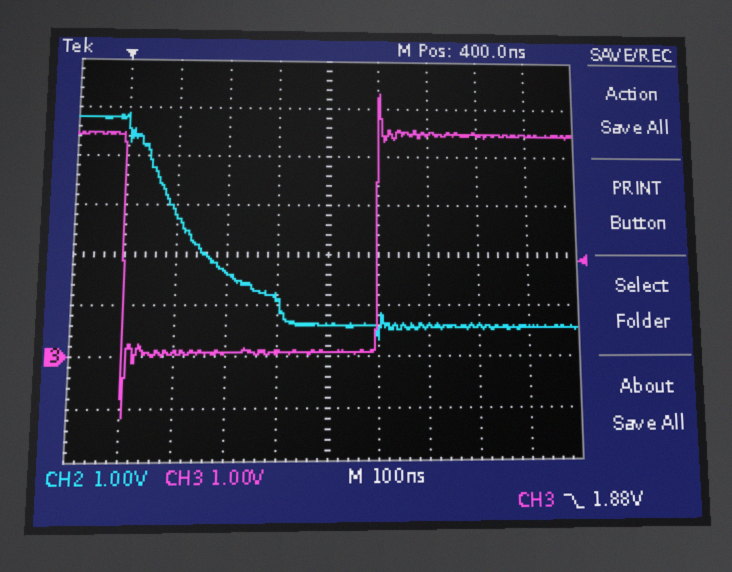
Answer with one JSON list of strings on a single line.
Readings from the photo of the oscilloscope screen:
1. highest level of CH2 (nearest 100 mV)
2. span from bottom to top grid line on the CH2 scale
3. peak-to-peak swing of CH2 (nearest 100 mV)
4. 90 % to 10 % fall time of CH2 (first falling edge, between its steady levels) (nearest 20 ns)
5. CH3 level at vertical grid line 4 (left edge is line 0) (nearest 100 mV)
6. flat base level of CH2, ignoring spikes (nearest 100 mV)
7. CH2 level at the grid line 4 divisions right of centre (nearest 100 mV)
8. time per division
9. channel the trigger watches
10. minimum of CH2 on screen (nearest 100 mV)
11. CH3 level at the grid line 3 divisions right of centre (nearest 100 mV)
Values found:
["4.9 V", "8 V", "4.6 V", "280 ns", "100 mV", "600 mV", "600 mV", "100 ns", "CH3", "300 mV", "4.5 V"]
